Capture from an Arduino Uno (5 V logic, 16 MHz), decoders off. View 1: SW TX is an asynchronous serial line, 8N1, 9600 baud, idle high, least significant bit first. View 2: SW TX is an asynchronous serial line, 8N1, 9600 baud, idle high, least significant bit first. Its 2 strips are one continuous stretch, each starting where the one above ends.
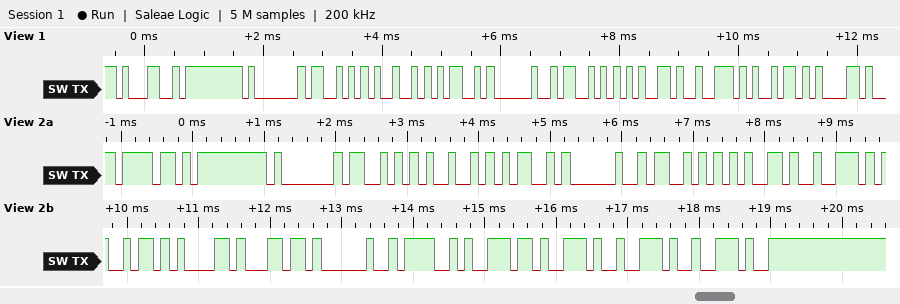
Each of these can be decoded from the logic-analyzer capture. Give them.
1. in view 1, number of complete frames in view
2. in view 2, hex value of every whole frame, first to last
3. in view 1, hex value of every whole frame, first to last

12
6F FF 01 53 49 4D 20 53 65 72 69 61 6C 20 4F 6E 2E 2E 2E
31 FF 01 53 49 4D 20 53 65 72 69 61
